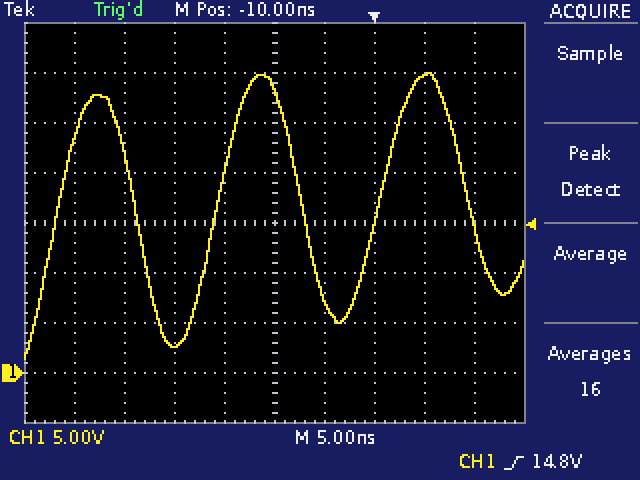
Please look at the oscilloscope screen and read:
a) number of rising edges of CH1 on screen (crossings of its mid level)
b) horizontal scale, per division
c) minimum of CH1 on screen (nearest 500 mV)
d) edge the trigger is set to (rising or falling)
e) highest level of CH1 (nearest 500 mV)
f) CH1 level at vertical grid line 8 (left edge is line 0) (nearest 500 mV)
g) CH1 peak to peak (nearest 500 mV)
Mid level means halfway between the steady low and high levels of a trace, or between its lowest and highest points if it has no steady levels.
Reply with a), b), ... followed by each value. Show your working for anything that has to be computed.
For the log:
a) 3
b) 5 ns
c) 1.5 V
d) rising
e) 30.0 V
f) 30.0 V
g) 30.0 V − (1.5 V) = 28.5 V
